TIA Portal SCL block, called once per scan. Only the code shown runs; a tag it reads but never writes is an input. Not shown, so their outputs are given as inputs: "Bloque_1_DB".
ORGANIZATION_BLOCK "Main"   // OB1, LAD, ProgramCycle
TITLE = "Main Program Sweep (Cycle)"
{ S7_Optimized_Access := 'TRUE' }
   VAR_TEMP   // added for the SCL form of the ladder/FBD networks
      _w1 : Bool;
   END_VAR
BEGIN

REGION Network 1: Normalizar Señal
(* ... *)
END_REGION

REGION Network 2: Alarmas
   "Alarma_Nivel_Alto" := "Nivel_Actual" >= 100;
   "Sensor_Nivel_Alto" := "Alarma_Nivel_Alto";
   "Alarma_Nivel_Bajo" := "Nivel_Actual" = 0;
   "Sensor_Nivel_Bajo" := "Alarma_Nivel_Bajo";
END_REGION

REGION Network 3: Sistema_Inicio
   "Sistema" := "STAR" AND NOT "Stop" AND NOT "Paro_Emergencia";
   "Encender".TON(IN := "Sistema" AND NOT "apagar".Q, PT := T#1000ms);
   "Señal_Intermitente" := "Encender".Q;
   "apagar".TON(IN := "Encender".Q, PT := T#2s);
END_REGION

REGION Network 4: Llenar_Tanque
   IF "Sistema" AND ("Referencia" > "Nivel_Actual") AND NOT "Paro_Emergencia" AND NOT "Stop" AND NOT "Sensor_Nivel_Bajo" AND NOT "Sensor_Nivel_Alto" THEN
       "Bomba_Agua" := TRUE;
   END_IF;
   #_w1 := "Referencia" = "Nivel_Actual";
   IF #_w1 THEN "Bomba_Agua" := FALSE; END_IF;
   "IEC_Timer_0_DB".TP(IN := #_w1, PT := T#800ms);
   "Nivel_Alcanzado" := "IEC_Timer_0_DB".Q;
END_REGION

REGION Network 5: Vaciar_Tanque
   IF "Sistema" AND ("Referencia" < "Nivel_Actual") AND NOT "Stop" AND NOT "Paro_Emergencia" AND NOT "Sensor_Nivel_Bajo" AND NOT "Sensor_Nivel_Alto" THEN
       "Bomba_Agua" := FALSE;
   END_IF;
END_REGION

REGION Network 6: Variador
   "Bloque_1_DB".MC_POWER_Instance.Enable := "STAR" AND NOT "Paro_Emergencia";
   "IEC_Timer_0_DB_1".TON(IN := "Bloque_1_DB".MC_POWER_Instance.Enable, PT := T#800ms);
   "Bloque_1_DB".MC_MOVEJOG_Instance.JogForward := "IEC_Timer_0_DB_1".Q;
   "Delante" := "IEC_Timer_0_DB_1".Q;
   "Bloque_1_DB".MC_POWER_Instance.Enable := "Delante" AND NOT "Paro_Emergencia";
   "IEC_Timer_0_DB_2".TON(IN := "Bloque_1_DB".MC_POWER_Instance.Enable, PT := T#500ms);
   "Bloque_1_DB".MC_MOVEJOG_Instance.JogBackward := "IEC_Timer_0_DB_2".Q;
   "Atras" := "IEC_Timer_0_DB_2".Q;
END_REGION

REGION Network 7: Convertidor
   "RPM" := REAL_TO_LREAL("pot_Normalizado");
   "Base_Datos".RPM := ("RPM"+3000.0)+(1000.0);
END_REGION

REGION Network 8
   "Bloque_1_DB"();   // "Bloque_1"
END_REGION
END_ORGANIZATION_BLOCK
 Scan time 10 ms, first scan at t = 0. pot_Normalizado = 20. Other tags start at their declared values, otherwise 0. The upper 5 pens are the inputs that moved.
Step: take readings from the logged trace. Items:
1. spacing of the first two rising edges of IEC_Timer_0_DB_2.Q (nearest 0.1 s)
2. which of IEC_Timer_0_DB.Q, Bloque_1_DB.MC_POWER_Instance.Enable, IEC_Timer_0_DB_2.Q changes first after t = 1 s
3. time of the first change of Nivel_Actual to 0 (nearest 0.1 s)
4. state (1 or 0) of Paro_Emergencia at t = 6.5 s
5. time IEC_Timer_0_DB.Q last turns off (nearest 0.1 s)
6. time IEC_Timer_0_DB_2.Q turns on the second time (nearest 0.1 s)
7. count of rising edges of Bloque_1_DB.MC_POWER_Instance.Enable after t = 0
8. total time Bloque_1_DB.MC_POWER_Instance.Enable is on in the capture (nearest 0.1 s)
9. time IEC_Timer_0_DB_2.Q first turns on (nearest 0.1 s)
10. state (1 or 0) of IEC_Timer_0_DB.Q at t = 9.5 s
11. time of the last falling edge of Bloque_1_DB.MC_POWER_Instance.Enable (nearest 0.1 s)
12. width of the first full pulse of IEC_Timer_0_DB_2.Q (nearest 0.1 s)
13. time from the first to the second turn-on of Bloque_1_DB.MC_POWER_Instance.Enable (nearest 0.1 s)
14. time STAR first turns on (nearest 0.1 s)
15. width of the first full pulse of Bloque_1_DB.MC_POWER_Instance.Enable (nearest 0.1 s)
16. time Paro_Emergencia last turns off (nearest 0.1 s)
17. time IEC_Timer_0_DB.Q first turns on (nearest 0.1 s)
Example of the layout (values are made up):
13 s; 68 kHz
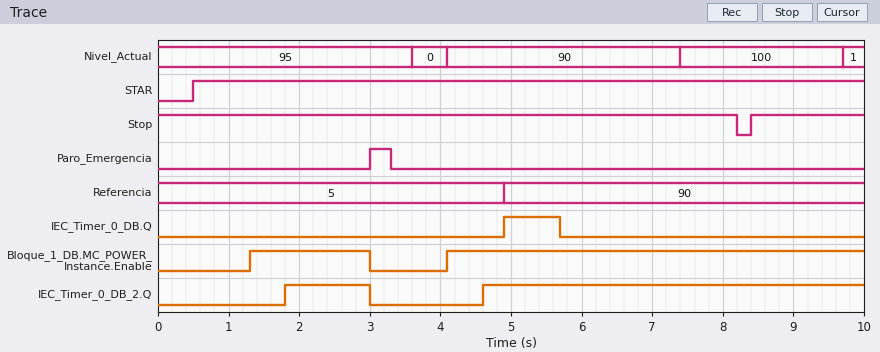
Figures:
2.8 s; Bloque_1_DB.MC_POWER_Instance.Enable; 3.6 s; 0; 5.7 s; 4.6 s; 2; 7.6 s; 1.8 s; 0; 3.0 s; 1.2 s; 2.8 s; 0.5 s; 1.7 s; 3.3 s; 4.9 s
